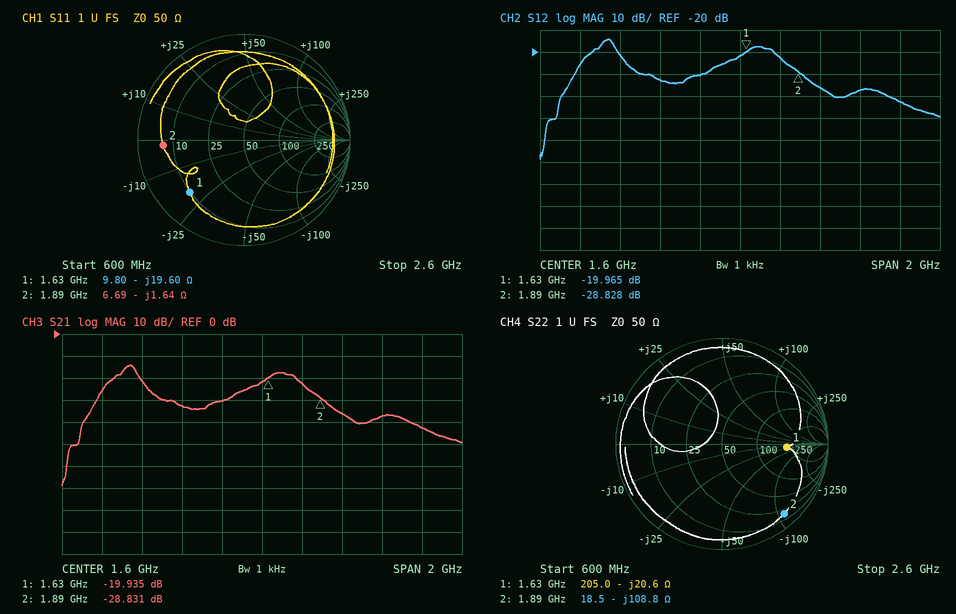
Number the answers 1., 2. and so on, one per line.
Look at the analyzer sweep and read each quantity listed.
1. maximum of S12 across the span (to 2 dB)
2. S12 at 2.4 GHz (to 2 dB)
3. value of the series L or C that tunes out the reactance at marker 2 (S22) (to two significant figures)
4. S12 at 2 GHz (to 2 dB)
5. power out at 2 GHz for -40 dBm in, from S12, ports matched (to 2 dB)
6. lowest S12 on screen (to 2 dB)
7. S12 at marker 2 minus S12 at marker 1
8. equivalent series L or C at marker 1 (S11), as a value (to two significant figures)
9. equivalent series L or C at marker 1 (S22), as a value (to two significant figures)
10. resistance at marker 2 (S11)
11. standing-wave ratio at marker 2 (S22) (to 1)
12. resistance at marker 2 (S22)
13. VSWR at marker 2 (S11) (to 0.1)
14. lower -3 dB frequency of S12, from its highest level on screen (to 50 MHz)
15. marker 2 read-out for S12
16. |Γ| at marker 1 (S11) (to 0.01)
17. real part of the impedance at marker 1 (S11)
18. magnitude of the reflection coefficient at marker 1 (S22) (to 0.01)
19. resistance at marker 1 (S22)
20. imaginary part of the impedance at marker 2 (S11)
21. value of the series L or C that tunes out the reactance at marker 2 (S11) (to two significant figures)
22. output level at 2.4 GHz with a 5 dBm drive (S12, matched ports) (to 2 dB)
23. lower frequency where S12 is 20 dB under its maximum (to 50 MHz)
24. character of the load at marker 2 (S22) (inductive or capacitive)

1. -14 dB
2. -42 dB
3. 9.2 nH
4. -36 dB
5. -76 dBm
6. -68 dB
7. -8.863 dB
8. 5.0 pF
9. 4.7 pF
10. 6.69 Ω
11. 16
12. 18.5 Ω
13. 7.5
14. 900 MHz
15. -28.828 dB
16. 0.71
17. 9.80 Ω
18. 0.61
19. 205.0 Ω
20. -1.64 Ω
21. 140 pH
22. -38 dBm
23. 750 MHz
24. capacitive
